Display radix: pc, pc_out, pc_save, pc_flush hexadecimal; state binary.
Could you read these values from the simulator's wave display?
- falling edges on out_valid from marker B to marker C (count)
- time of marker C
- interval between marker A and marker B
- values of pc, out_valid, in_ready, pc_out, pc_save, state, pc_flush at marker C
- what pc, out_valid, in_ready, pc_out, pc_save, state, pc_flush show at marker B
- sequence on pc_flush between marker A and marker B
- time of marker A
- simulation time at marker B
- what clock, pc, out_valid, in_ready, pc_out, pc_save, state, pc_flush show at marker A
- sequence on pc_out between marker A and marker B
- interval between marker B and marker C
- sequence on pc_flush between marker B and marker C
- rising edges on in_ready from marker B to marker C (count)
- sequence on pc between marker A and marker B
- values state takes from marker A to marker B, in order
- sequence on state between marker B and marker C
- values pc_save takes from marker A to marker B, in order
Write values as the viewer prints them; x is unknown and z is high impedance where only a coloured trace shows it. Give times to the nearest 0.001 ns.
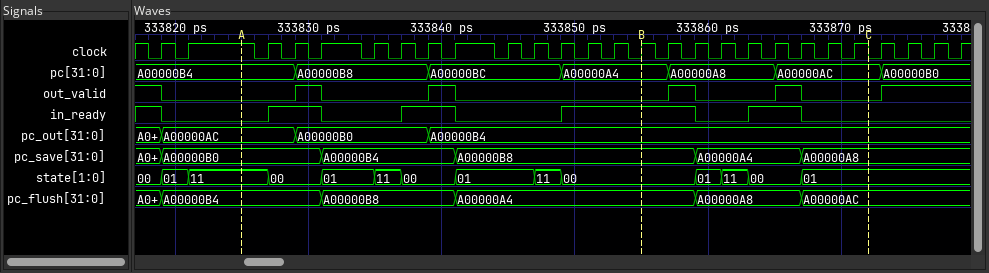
2
333.872 ns
0.03 ns
pc=A00000AC, out_valid=0, in_ready=0, pc_out=A00000B4, pc_save=A00000A8, state=01, pc_flush=A00000AC
pc=A00000A4, out_valid=0, in_ready=1, pc_out=A00000B4, pc_save=A00000B8, state=00, pc_flush=A00000A4
A00000B4, A00000B8, A00000A4
333.825 ns
333.855 ns
clock=1, pc=A00000B4, out_valid=0, in_ready=0, pc_out=A00000AC, pc_save=A00000B0, state=11, pc_flush=A00000B4
A00000AC, A00000B0, A00000B4
0.017 ns
A00000A4, A00000A8, A00000AC
1
A00000B4, A00000B8, A00000BC, A00000A4
11, 00, 01, 11, 00, 01, 11, 00
00, 01, 11, 00, 01
A00000B0, A00000B4, A00000B8
